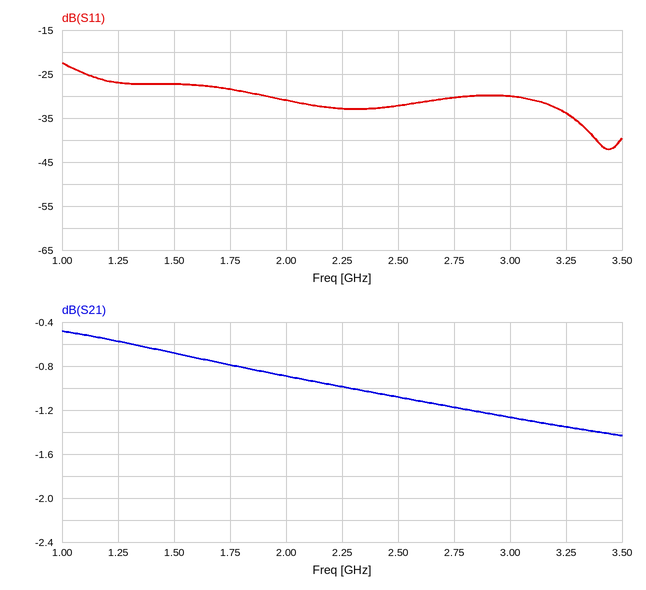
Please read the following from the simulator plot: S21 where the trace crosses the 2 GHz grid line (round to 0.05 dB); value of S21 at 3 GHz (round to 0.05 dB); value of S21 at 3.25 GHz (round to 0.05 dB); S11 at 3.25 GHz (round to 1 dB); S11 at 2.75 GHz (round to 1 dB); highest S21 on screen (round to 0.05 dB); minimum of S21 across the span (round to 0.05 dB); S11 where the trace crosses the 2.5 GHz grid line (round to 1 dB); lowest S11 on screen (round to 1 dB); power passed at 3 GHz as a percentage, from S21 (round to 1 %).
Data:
-0.90 dB
-1.25 dB
-1.35 dB
-34 dB
-30 dB
-0.50 dB
-1.45 dB
-32 dB
-42 dB
75 %
